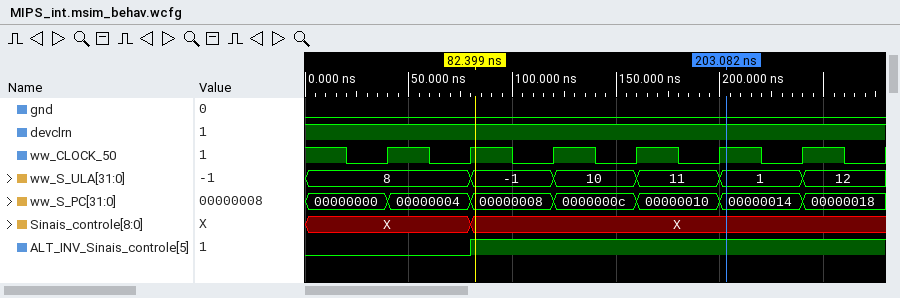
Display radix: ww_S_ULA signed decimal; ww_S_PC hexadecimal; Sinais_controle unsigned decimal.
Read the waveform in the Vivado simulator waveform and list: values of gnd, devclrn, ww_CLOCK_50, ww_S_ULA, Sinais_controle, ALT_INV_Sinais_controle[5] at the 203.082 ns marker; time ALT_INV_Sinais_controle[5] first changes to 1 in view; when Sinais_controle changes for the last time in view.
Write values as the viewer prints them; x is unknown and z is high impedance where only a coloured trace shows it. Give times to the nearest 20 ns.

gnd=0, devclrn=1, ww_CLOCK_50=1, ww_S_ULA=1, Sinais_controle=X, ALT_INV_Sinais_controle[5]=1
80 ns
80 ns
